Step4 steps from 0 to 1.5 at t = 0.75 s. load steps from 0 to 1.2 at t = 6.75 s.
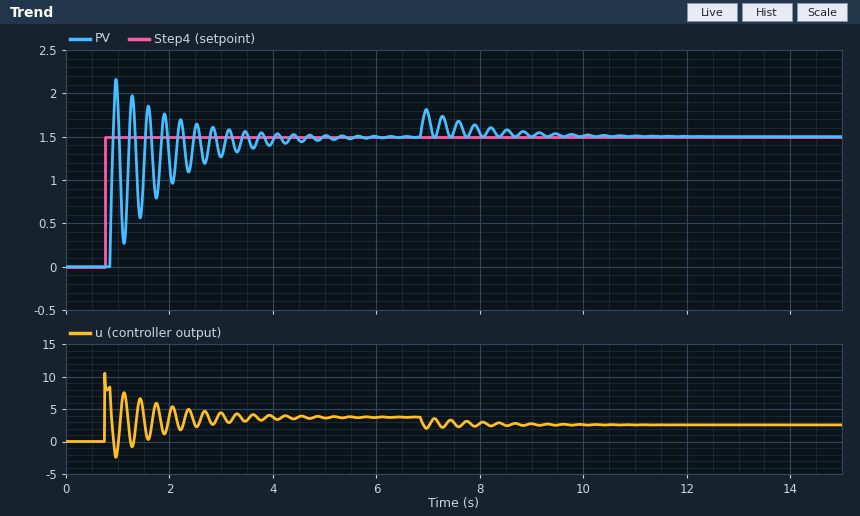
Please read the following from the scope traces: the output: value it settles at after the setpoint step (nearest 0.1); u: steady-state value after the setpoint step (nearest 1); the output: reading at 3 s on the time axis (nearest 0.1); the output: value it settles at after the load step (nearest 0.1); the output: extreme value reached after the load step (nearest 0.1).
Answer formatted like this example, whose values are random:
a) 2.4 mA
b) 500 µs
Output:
a) 1.5
b) 4
c) 1.3
d) 1.5
e) 1.8
